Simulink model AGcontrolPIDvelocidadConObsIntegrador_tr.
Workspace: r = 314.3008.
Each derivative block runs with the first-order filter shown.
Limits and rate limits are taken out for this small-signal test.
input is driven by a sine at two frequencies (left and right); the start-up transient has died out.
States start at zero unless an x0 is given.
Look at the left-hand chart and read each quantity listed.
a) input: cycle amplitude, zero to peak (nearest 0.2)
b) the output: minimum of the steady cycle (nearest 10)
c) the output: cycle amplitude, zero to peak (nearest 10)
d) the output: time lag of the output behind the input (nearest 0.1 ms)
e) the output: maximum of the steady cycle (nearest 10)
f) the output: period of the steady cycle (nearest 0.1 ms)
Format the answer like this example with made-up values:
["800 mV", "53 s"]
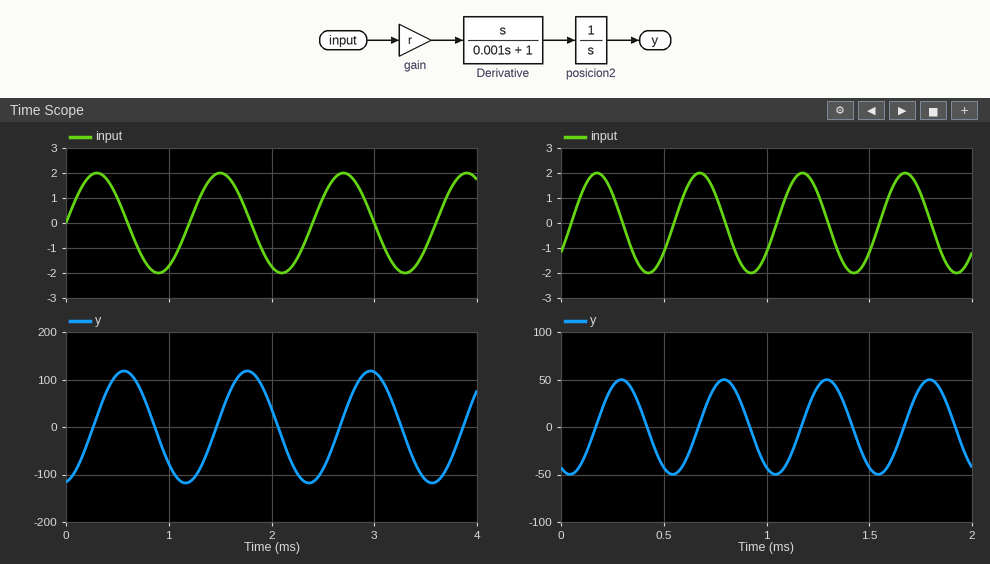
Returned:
["2.0", "-120", "120", "0.3 ms", "120", "1.2 ms"]
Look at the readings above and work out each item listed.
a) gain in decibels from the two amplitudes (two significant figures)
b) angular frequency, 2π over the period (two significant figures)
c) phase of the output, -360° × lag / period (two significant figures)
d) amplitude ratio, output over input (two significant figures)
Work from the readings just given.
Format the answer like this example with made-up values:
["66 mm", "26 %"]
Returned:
["36 dB", "5.2 rad/ms", "-90°", "60"]
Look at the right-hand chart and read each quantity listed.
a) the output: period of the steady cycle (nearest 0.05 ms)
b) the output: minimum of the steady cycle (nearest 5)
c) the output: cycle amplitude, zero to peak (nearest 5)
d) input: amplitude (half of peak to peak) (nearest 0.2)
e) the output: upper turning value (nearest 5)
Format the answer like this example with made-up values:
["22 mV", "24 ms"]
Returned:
["0.50 ms", "-50", "50", "2.0", "50"]
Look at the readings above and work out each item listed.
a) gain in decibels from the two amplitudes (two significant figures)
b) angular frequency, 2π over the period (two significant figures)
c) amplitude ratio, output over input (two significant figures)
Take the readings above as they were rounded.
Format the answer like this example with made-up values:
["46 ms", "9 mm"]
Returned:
["28 dB", "13 rad/ms", "25"]
